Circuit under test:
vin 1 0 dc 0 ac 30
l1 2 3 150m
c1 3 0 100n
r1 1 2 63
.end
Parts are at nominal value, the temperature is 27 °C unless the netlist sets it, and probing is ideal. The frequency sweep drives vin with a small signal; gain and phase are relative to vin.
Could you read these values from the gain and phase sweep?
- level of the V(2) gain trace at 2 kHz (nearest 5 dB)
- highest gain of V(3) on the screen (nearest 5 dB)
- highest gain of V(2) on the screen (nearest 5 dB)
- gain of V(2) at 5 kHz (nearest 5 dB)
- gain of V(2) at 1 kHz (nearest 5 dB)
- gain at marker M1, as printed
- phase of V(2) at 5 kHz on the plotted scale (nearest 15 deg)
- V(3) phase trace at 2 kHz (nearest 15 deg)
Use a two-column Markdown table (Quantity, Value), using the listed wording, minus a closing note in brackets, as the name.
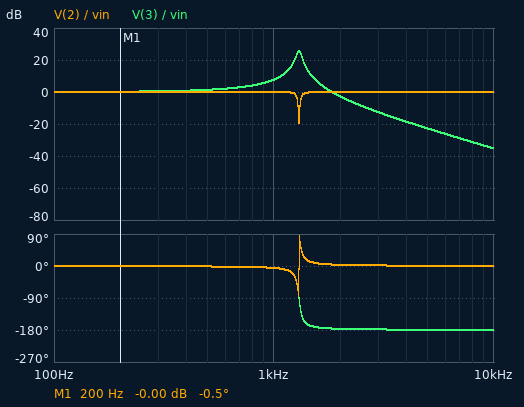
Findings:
| Quantity | Value |
|---|---|
| level of the V(2) gain trace at 2 kHz | 0 dB |
| highest gain of V(3) on the screen | 25 dB |
| highest gain of V(2) on the screen | 0 dB |
| gain of V(2) at 5 kHz | 0 dB |
| gain of V(2) at 1 kHz | 0 dB |
| gain at marker M1, as printed | -0.00 dB |
| phase of V(2) at 5 kHz on the plotted scale | 0 deg |
| V(3) phase trace at 2 kHz | -180 deg |
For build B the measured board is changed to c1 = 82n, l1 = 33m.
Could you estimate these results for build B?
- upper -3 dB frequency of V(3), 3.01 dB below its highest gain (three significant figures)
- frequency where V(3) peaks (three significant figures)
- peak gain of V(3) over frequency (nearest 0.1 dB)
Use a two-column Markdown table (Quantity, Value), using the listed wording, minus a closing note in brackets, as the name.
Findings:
| Quantity | Value |
|---|---|
| upper -3 dB frequency of V(3), 3.01 dB below its highest gain | 3.20 kHz |
| frequency where V(3) peaks | 3.05 kHz |
| peak gain of V(3) over frequency | 20.1 dB |
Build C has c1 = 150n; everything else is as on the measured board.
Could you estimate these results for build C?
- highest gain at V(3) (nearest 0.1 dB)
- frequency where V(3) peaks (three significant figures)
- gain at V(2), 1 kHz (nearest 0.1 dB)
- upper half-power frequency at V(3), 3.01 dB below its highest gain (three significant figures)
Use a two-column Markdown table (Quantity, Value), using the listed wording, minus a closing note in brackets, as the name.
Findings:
| Quantity | Value |
|---|---|
| highest gain at V(3) | 24.0 dB |
| frequency where V(3) peaks | 1.06 kHz |
| gain at V(2), 1 kHz | -1.1 dB |
| upper half-power frequency at V(3), 3.01 dB below its highest gain | 1.09 kHz |
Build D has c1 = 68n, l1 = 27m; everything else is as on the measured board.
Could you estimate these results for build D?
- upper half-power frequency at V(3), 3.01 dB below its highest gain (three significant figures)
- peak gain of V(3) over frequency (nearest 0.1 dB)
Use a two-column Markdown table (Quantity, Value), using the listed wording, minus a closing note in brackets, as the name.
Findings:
| Quantity | Value |
|---|---|
| upper half-power frequency at V(3), 3.01 dB below its highest gain | 3.89 kHz |
| peak gain of V(3) over frequency | 20.0 dB |
